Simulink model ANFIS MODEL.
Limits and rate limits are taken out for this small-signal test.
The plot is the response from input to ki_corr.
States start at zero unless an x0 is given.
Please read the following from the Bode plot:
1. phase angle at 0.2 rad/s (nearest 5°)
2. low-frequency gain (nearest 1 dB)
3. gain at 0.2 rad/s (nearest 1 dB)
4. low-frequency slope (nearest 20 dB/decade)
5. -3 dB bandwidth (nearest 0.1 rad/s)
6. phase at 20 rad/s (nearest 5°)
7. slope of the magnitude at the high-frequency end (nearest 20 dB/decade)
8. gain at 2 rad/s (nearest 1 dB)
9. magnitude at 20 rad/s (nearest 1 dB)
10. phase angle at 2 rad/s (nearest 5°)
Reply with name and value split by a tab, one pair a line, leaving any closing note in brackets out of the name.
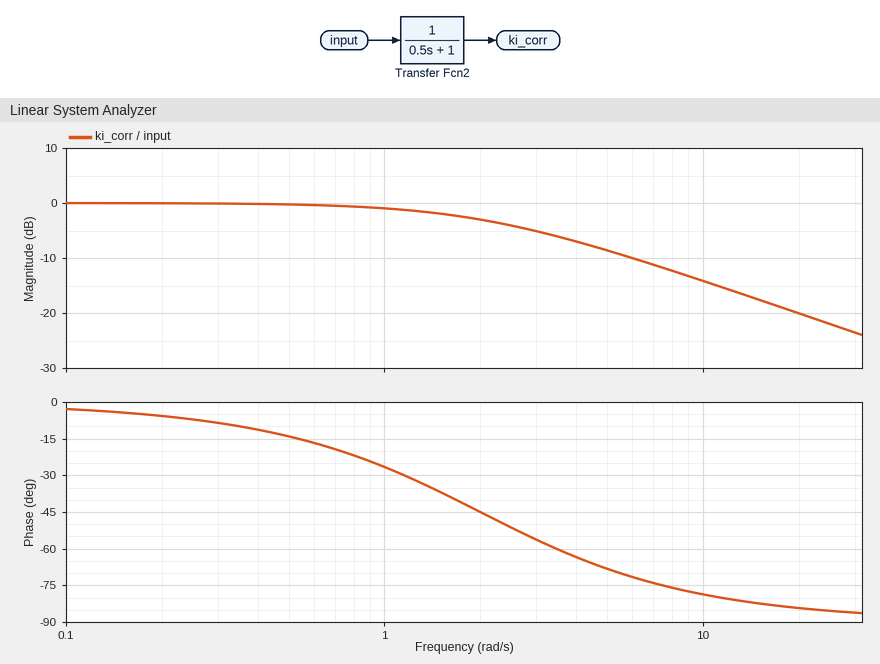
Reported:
phase angle at 0.2 rad/s	-5°
low-frequency gain	0 dB
gain at 0.2 rad/s	0 dB
low-frequency slope	0 dB/decade
-3 dB bandwidth	2.0 rad/s
phase at 20 rad/s	-85°
slope of the magnitude at the high-frequency end	-20 dB/decade
gain at 2 rad/s	-3 dB
magnitude at 20 rad/s	-20 dB
phase angle at 2 rad/s	-45°
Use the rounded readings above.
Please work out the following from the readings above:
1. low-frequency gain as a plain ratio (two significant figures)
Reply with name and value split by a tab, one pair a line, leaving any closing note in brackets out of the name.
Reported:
low-frequency gain as a plain ratio	1.0
